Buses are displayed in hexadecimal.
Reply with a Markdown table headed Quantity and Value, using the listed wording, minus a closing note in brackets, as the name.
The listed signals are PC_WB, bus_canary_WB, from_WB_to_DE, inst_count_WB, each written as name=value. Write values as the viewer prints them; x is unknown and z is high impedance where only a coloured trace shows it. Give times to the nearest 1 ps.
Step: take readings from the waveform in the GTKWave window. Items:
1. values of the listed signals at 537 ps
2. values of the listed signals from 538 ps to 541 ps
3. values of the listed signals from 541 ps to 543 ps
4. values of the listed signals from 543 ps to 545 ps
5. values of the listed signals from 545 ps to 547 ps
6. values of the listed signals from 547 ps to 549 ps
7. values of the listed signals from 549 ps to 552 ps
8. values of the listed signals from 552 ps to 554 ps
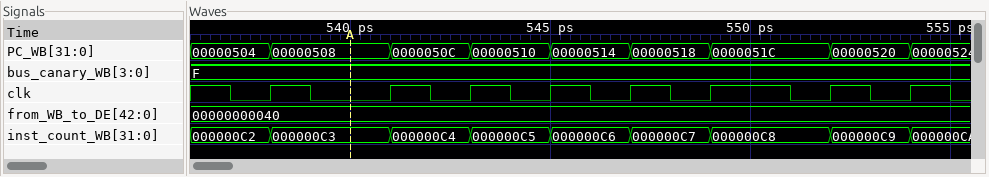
| Quantity | Value |
|---|---|
| values of the listed signals at 537 ps | PC_WB=00000504, bus_canary_WB=F, from_WB_to_DE=00000000040, inst_count_WB=000000C2 |
| values of the listed signals from 538 ps to 541 ps | PC_WB=00000508, bus_canary_WB=F, from_WB_to_DE=00000000040, inst_count_WB=000000C3 |
| values of the listed signals from 541 ps to 543 ps | PC_WB=0000050C, bus_canary_WB=F, from_WB_to_DE=00000000040, inst_count_WB=000000C4 |
| values of the listed signals from 543 ps to 545 ps | PC_WB=00000510, bus_canary_WB=F, from_WB_to_DE=00000000040, inst_count_WB=000000C5 |
| values of the listed signals from 545 ps to 547 ps | PC_WB=00000514, bus_canary_WB=F, from_WB_to_DE=00000000040, inst_count_WB=000000C6 |
| values of the listed signals from 547 ps to 549 ps | PC_WB=00000518, bus_canary_WB=F, from_WB_to_DE=00000000040, inst_count_WB=000000C7 |
| values of the listed signals from 549 ps to 552 ps | PC_WB=0000051C, bus_canary_WB=F, from_WB_to_DE=00000000040, inst_count_WB=000000C8 |
| values of the listed signals from 552 ps to 554 ps | PC_WB=00000520, bus_canary_WB=F, from_WB_to_DE=00000000040, inst_count_WB=000000C9 |
